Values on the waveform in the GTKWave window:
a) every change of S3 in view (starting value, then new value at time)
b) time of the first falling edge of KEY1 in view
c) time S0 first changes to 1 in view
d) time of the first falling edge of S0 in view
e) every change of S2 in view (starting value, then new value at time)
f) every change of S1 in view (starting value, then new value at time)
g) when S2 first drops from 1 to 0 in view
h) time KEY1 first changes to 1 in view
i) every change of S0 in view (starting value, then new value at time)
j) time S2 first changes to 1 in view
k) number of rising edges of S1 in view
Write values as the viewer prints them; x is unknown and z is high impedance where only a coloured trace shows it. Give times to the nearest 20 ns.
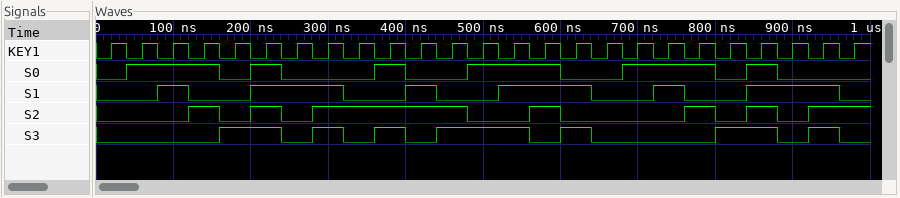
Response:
0, 1 at 160 ns, 0 at 240 ns, 1 at 280 ns, 0 at 320 ns, 1 at 360 ns, 0 at 400 ns, 1 at 440 ns, 0 at 560 ns, 1 at 600 ns, 0 at 640 ns, 1 at 800 ns, 0 at 880 ns, 1 at 920 ns, 0 at 960 ns
40 ns
40 ns
160 ns
0, 1 at 120 ns, 0 at 160 ns, 1 at 200 ns, 0 at 240 ns, 1 at 280 ns, 0 at 480 ns, 1 at 560 ns, 0 at 600 ns, 1 at 760 ns, 0 at 800 ns, 1 at 840 ns, 0 at 880 ns, 1 at 920 ns
0, 1 at 80 ns, 0 at 120 ns, 1 at 200 ns, 0 at 320 ns, 1 at 400 ns, 0 at 440 ns, 1 at 520 ns, 0 at 640 ns, 1 at 720 ns, 0 at 760 ns, 1 at 840 ns, 0 at 960 ns
160 ns
20 ns
0, 1 at 40 ns, 0 at 160 ns, 1 at 200 ns, 0 at 240 ns, 1 at 360 ns, 0 at 400 ns, 1 at 480 ns, 0 at 600 ns, 1 at 680 ns, 0 at 800 ns, 1 at 840 ns, 0 at 880 ns
120 ns
6
